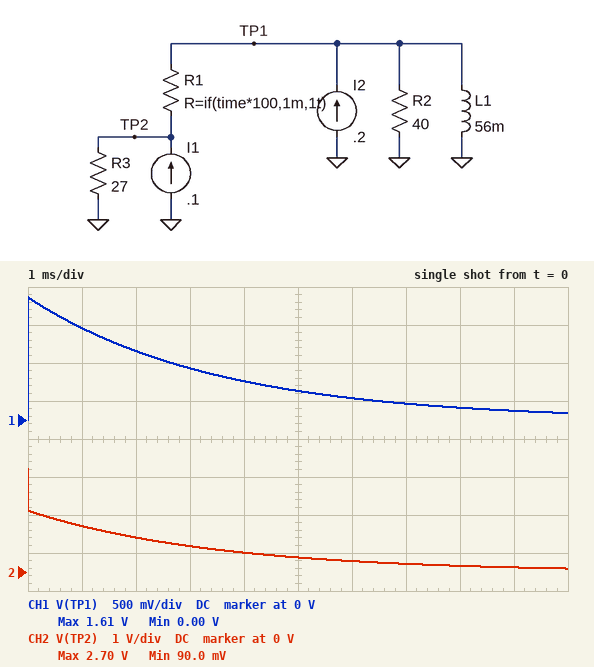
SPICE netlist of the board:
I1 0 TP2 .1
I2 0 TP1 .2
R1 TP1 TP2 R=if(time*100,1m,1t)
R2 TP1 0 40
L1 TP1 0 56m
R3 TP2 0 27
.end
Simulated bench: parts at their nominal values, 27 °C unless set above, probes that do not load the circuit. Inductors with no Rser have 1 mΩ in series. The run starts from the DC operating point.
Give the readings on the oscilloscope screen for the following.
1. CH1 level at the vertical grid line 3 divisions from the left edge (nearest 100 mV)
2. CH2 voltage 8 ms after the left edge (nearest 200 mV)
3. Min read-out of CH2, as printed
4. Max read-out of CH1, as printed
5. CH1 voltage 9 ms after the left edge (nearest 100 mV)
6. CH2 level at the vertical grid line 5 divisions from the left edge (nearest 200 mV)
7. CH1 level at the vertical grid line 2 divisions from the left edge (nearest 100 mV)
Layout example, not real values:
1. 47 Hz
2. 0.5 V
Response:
1. 700 mV
2. 200 mV
3. 90.0 mV
4. 1.61 V
5. 100 mV
6. 400 mV
7. 900 mV
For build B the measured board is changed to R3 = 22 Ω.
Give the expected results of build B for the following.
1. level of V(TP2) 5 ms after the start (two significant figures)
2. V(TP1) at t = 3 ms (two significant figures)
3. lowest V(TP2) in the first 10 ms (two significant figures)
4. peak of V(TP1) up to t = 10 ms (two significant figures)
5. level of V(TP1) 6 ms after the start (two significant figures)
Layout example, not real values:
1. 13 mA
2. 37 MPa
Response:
1. 400 mV
2. 660 mV
3. 110 mV
4. 1.4 V
5. 310 mV
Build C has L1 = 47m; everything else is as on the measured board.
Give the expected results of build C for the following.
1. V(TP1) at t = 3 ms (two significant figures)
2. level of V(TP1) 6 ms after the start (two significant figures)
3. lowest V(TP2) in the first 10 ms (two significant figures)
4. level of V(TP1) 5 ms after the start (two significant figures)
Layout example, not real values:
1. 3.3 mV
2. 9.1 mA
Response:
1. 580 mV
2. 210 mV
3. 53 mV
4. 290 mV
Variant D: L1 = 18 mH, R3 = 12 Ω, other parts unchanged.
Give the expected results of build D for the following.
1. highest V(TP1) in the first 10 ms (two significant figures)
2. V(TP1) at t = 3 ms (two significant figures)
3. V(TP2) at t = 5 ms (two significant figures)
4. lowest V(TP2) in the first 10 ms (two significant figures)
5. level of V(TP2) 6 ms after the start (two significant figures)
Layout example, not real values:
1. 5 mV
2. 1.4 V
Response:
1. 920 mV
2. 200 mV
3. 71 mV
4. 5.9 mV
5. 43 mV
